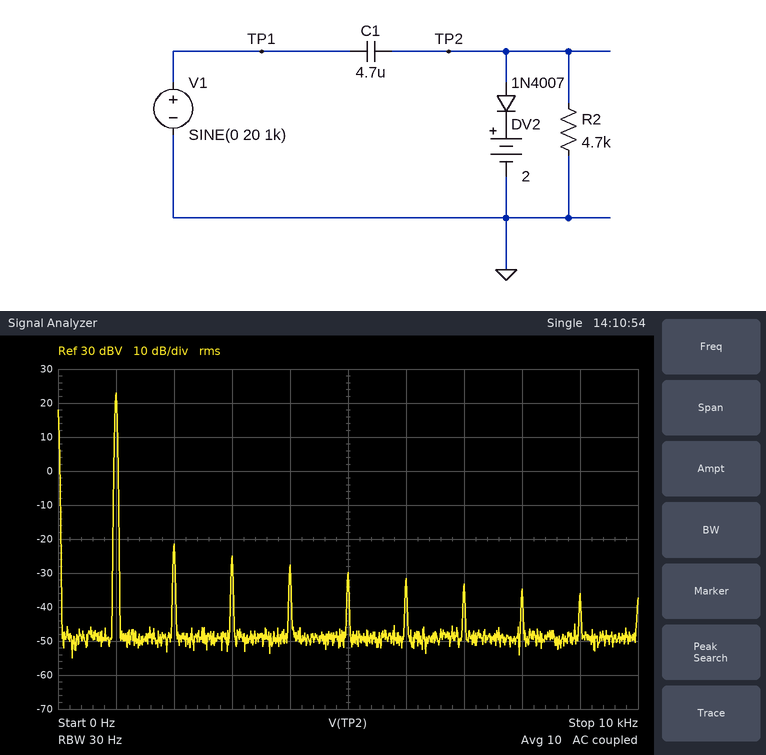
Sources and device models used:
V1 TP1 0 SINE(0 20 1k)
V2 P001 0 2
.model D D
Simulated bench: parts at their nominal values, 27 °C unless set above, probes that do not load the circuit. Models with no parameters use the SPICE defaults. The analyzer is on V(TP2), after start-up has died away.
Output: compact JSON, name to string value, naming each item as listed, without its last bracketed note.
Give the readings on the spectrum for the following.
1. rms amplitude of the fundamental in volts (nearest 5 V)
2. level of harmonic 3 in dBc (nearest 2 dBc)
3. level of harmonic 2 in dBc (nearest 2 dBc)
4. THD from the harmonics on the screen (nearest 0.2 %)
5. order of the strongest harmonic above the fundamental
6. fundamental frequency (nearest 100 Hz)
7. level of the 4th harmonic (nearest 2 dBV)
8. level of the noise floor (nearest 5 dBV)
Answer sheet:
{"rms amplitude of the fundamental in volts": "15 V", "level of harmonic 3 in dBc": "-48 dBc", "level of harmonic 2 in dBc": "-44 dBc", "THD from the harmonics on the screen": "0.8 %", "order of the strongest harmonic above the fundamental": "2", "fundamental frequency": "1.0 kHz", "level of the 4th harmonic": "-28 dBV", "level of the noise floor": "-50 dBV"}
